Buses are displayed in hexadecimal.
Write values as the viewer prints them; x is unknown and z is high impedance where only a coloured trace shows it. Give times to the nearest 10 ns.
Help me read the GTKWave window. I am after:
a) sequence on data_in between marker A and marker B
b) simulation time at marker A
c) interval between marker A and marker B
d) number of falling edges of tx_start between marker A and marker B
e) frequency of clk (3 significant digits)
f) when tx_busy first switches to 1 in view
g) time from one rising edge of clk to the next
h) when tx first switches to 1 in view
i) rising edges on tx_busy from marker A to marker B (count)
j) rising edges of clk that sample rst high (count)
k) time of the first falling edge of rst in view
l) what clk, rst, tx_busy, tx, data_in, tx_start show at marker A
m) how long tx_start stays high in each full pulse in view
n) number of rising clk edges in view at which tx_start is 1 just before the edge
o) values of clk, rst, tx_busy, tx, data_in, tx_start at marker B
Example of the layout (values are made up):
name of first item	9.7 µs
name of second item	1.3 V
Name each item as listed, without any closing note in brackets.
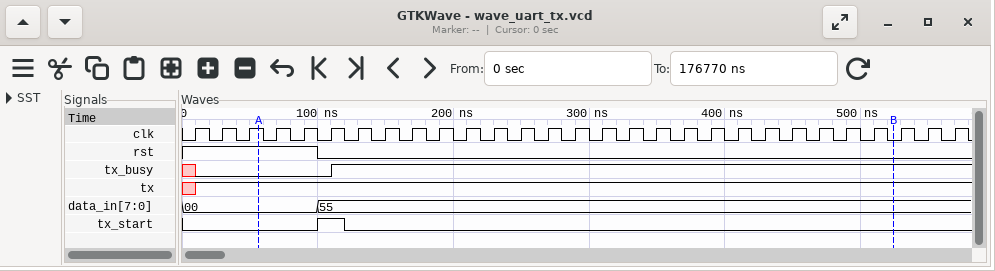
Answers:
sequence on data_in between marker A and marker B	00, 55
simulation time at marker A	60 ns
interval between marker A and marker B	470 ns
number of falling edges of tx_start between marker A and marker B	1
frequency of clk	50.0 MHz
when tx_busy first switches to 1 in view	110 ns
time from one rising edge of clk to the next	20 ns
when tx first switches to 1 in view	10 ns
rising edges on tx_busy from marker A to marker B	1
rising edges of clk that sample rst high	5
time of the first falling edge of rst in view	100 ns
what clk, rst, tx_busy, tx, data_in, tx_start show at marker A	clk=1, rst=1, tx_busy=0, tx=1, data_in=00, tx_start=0
how long tx_start stays high in each full pulse in view	20 ns
number of rising clk edges in view at which tx_start is 1 just before the edge	1
values of clk, rst, tx_busy, tx, data_in, tx_start at marker B	clk=0, rst=0, tx_busy=1, tx=1, data_in=55, tx_start=0
